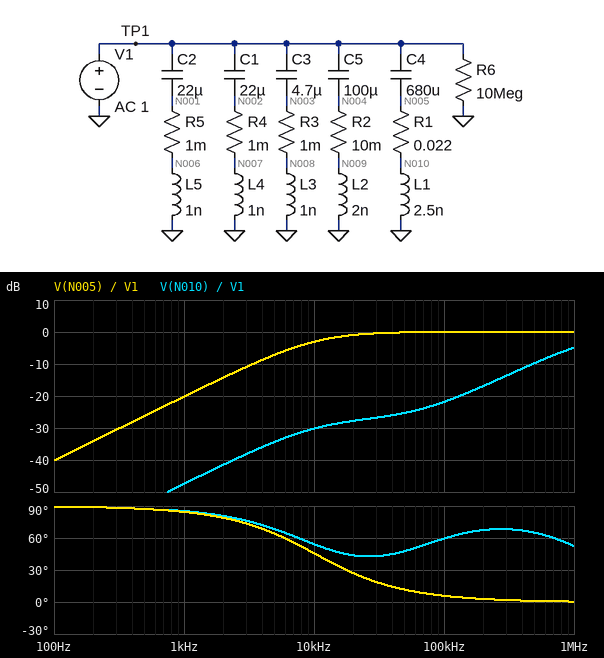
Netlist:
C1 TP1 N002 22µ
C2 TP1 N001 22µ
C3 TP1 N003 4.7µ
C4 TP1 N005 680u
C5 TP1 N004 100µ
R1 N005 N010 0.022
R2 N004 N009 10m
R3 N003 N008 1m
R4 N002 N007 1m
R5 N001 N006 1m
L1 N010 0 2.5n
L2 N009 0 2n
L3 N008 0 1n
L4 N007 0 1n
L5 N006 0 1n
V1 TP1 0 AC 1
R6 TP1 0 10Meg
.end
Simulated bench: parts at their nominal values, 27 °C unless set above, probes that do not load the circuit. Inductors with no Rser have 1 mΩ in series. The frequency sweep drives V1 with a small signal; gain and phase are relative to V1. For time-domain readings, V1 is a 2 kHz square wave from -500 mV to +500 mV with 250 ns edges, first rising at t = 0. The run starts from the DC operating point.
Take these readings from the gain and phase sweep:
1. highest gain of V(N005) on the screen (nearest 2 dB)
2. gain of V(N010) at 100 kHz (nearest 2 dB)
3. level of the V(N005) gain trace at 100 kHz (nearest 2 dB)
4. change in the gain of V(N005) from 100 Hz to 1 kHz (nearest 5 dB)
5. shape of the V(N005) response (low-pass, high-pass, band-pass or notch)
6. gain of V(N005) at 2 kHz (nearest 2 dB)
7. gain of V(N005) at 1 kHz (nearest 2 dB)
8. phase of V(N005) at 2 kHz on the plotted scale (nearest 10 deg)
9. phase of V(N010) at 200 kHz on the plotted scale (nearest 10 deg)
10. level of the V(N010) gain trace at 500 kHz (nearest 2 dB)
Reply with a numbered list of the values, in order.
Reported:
1. 0 dB
2. -22 dB
3. 0 dB
4. 20 dB
5. high-pass
6. -14 dB
7. -20 dB
8. 80 deg
9. 70 deg
10. -10 dB
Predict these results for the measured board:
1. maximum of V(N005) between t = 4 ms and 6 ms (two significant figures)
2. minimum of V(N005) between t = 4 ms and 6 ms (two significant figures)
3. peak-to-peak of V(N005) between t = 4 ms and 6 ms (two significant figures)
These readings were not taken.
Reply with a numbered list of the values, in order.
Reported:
1. 1.0 V
2. -1.0 V
3. 2.0 V
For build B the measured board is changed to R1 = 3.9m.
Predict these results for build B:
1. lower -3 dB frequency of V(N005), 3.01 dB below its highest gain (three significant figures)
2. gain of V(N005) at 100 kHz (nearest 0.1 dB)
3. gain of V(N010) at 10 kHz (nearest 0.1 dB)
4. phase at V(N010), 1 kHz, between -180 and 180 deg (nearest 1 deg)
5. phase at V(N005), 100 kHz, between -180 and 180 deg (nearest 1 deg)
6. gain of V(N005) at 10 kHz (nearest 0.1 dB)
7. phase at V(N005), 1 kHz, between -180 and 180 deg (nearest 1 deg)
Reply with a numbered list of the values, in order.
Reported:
1. 48.6 kHz
2. 0.3 dB
3. -27.4 dB
4. 90 deg
5. 27 deg
6. -13.7 dB
7. 89 deg
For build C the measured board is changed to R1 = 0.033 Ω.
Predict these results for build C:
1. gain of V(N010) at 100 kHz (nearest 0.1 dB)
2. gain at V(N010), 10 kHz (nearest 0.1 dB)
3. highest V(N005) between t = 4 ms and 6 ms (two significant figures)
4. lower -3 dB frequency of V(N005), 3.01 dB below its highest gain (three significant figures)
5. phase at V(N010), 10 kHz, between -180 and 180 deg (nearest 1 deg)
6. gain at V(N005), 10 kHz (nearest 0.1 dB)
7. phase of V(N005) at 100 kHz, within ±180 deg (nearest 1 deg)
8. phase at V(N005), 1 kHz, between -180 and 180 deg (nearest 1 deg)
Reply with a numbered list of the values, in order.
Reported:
1. -25.2 dB
2. -32.2 dB
3. 1.0 V
4. 6.90 kHz
5. 43 deg
6. -1.7 dB
7. 4 deg
8. 82 deg
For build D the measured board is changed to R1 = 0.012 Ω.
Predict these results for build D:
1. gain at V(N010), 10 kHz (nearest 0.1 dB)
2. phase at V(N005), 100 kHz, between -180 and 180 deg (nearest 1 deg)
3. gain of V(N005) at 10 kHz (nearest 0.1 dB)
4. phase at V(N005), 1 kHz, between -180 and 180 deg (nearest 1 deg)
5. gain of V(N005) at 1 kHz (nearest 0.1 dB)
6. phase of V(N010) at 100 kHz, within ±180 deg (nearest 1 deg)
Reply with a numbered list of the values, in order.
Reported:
1. -28.4 dB
2. 10 deg
3. -6.2 dB
4. 87 deg
5. -25.1 dB
6. 61 deg
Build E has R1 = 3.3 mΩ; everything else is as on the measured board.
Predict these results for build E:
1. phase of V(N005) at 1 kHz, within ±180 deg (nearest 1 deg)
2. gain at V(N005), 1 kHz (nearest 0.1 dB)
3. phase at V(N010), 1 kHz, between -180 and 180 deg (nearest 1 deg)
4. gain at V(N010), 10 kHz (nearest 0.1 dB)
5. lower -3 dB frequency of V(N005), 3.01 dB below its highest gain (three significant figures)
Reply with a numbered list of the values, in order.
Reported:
1. 89 deg
2. -34.7 dB
3. 90 deg
4. -27.4 dB
5. 54.6 kHz
